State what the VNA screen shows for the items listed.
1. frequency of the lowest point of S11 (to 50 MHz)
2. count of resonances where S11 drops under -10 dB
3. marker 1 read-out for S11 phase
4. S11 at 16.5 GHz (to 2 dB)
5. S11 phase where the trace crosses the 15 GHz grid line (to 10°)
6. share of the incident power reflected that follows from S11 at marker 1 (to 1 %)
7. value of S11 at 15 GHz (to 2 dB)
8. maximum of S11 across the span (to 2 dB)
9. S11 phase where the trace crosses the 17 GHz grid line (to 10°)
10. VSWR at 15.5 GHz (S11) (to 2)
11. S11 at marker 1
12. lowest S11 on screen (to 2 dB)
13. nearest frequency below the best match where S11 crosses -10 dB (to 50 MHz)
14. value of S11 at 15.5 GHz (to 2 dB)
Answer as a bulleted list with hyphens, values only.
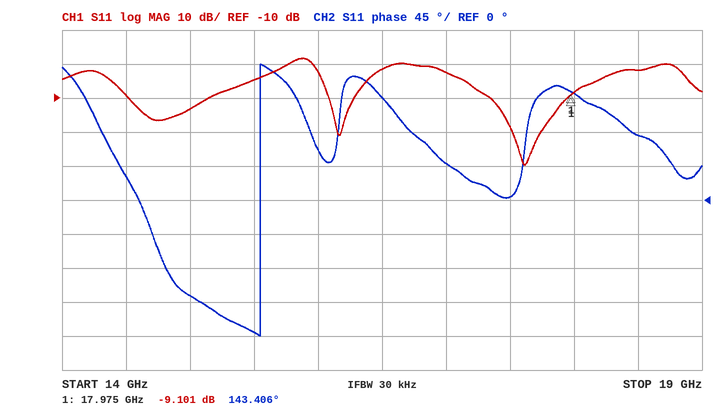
- 17.60 GHz
- 3
- 143.406°
- -2 dB
- -130°
- 12 %
- -14 dB
- 2 dB
- 50°
- 4
- -9.101 dB
- -30 dB
- 17.35 GHz
- -4 dB
